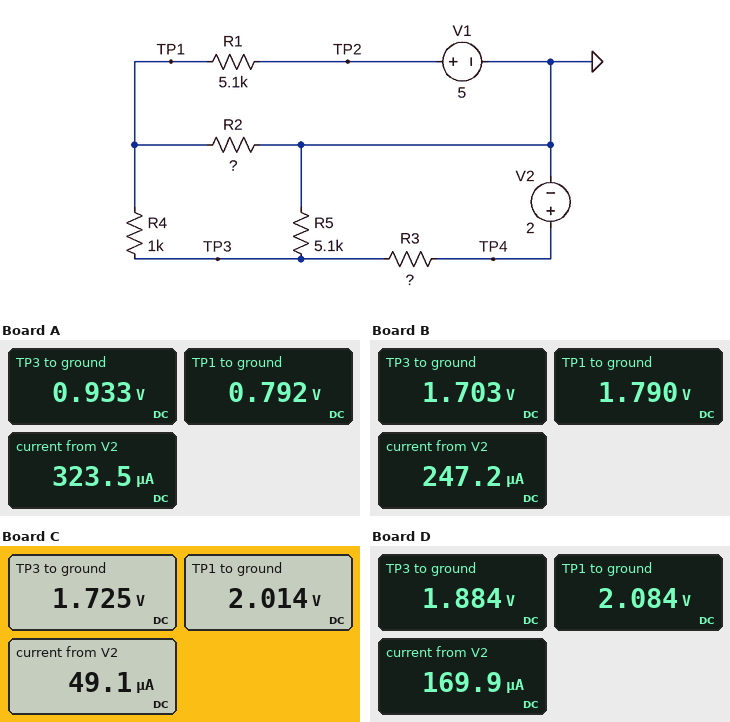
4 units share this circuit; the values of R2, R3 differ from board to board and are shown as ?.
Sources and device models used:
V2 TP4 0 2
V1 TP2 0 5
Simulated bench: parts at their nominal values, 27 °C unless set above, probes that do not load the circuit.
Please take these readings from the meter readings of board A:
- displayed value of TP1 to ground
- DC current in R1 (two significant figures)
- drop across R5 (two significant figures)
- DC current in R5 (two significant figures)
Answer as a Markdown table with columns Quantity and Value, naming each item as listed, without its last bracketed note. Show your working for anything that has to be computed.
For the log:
| Quantity | Value |
|---|---|
| displayed value of TP1 to ground | 0.792 V |
| DC current in R1 | (5 V - 792 mV) / 5.1 kΩ = 830 µA |
| drop across R5 | 933 mV = 930 mV |
| DC current in R5 | (933 mV) / 5.1 kΩ = 180 µA |
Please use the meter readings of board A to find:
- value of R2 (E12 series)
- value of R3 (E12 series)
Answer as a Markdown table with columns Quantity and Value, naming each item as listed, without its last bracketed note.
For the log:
| Quantity | Value |
|---|---|
| value of R2 | 820 Ω |
| value of R3 | 3.3 kΩ |
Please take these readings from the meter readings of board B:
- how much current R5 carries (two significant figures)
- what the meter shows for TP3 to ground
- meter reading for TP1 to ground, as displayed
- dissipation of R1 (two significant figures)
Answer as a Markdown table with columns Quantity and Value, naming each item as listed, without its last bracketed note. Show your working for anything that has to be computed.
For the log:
| Quantity | Value |
|---|---|
| how much current R5 carries | (1.703 V) / 5.1 kΩ = 330 µA |
| what the meter shows for TP3 to ground | 1.703 V |
| meter reading for TP1 to ground, as displayed | 1.790 V |
| dissipation of R1 | (5 V - 1.79 V)^2 / 5.1 kΩ = 2.0 mW |
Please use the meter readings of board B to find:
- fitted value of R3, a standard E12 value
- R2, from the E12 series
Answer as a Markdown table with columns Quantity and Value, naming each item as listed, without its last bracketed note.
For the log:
| Quantity | Value |
|---|---|
| fitted value of R3, a standard E12 value | 1.2 kΩ |
| R2, from the E12 series | 3.3 kΩ |
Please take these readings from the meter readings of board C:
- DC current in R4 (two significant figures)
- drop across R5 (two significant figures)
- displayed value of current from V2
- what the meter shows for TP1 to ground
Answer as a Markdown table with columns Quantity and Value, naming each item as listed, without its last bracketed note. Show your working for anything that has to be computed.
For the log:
| Quantity | Value |
|---|---|
| DC current in R4 | (2.014 V - 1.725 V) / 1 kΩ = 290 µA |
| drop across R5 | 1.725 V = 1.7 V |
| displayed value of current from V2 | 49.1 µA |
| what the meter shows for TP1 to ground | 2.014 V |
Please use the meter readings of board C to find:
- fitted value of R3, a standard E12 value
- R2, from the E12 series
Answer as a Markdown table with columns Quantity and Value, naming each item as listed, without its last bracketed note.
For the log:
| Quantity | Value |
|---|---|
| fitted value of R3, a standard E12 value | 5.6 kΩ |
| R2, from the E12 series | 6.8 kΩ |
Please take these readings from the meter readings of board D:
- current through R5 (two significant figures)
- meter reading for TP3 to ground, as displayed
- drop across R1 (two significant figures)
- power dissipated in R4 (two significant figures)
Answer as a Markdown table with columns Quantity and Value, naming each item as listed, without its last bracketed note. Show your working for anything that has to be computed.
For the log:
| Quantity | Value |
|---|---|
| current through R5 | (1.884 V) / 5.1 kΩ = 370 µA |
| meter reading for TP3 to ground, as displayed | 1.884 V |
| drop across R1 | 5 V - 2.084 V = 2.9 V |
| power dissipated in R4 | (2.084 V - 1.884 V)^2 / 1 kΩ = 40 µW |
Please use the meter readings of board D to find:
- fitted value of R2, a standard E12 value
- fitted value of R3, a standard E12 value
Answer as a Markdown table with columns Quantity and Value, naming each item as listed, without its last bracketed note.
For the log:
| Quantity | Value |
|---|---|
| fitted value of R2, a standard E12 value | 5.6 kΩ |
| fitted value of R3, a standard E12 value | 680 Ω |
